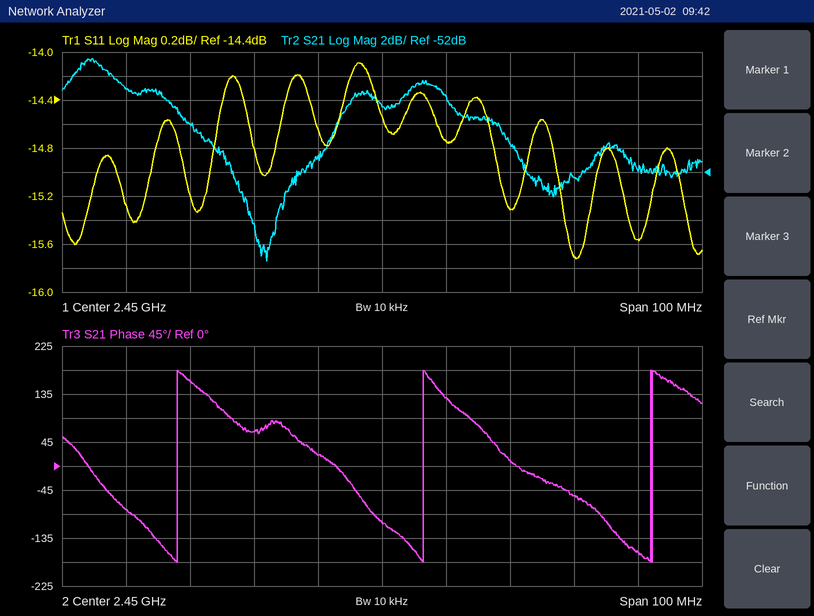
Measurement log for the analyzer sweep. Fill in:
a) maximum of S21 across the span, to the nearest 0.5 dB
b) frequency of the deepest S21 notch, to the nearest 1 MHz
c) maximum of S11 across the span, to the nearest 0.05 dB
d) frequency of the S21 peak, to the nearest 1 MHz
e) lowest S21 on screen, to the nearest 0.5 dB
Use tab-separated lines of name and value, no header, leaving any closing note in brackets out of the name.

maximum of S21 across the span, to the nearest 0.5 dB	-42.5 dB
frequency of the deepest S21 notch, to the nearest 1 MHz	2.432 GHz
maximum of S11 across the span, to the nearest 0.05 dB	-14.10 dB
frequency of the S21 peak, to the nearest 1 MHz	2.405 GHz
lowest S21 on screen, to the nearest 0.5 dB	-59.5 dB
